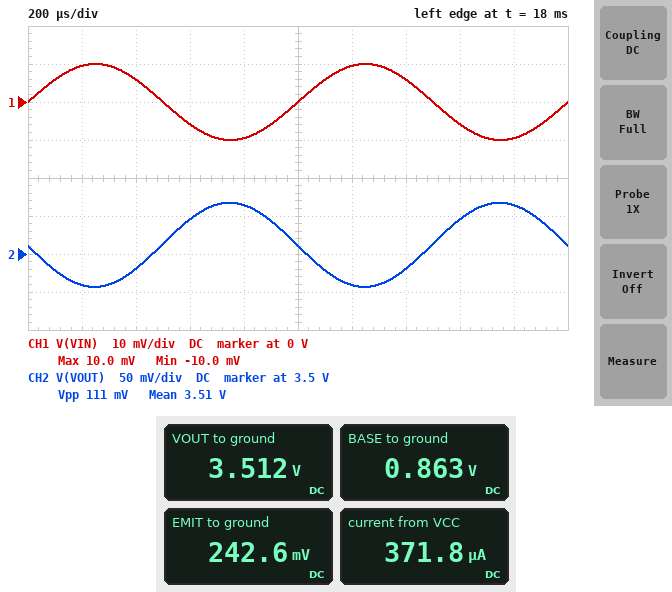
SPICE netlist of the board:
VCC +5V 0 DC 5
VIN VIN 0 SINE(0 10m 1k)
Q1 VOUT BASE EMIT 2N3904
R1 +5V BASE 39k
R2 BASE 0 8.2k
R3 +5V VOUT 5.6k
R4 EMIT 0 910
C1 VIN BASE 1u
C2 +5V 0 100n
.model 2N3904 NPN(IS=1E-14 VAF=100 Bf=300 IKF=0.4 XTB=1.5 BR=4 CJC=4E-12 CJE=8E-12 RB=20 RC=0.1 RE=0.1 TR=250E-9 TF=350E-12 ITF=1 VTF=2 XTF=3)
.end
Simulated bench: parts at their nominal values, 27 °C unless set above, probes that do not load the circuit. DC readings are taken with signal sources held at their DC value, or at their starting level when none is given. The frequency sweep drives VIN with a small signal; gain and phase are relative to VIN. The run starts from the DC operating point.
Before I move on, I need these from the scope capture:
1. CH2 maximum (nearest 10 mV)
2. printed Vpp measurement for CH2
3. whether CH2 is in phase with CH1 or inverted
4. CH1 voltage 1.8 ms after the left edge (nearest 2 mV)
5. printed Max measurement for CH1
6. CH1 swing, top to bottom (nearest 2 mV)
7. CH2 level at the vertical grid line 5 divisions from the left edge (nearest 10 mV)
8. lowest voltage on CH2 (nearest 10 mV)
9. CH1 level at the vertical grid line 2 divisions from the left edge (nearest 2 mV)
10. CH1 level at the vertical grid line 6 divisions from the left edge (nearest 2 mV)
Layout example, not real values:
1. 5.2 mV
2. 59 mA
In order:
1. 3.57 V
2. 111 mV
3. inverted
4. -10 mV
5. 10.0 mV
6. 20 mV
7. 3.51 V
8. 3.46 V
9. 6 mV
10. 10 mV
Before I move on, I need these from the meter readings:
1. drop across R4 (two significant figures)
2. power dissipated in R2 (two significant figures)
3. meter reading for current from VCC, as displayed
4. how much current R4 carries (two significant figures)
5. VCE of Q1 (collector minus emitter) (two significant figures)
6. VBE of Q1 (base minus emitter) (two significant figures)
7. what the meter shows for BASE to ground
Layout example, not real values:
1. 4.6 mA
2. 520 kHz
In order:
1. 240 mV
2. 91 µW
3. 371.8 µA
4. 270 µA
5. 3.3 V
6. 620 mV
7. 0.863 V
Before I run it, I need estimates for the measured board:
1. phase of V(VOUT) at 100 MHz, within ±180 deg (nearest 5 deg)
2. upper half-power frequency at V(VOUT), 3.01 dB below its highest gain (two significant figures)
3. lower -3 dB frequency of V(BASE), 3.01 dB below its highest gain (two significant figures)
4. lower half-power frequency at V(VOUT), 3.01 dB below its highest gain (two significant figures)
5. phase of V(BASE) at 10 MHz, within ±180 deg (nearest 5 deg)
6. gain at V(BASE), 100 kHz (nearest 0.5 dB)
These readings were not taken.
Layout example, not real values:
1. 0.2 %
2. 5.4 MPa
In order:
1. 20 deg
2. 12 MHz
3. 24 Hz
4. 24 Hz
5. 0 deg
6. 0 dB
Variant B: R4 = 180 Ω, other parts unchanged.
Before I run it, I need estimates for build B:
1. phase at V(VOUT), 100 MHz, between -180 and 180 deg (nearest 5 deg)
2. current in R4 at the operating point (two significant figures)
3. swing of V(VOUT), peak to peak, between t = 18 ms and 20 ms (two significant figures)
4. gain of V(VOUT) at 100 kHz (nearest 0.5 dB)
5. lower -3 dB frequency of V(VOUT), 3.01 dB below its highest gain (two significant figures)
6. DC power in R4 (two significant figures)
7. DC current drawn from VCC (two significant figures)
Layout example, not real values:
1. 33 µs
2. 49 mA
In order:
1. 0 deg
2. 860 µA
3. 310 mV
4. 17.0 dB
5. 350 Hz
6. 130 µW
7. 960 µA
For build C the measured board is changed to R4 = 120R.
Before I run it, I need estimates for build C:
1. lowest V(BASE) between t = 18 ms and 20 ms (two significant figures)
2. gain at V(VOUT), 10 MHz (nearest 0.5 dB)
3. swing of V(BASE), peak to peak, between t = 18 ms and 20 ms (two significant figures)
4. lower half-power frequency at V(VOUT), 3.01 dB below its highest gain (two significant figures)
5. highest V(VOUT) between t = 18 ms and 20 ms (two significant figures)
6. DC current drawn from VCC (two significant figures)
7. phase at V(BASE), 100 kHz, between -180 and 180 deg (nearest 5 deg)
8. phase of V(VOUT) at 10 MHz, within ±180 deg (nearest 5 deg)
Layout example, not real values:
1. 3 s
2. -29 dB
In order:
1. 750 mV
2. -1.0 dB
3. 19 mV
4. 520 Hz
5. 460 mV
6. 970 µA
7. 0 deg
8. 10 deg
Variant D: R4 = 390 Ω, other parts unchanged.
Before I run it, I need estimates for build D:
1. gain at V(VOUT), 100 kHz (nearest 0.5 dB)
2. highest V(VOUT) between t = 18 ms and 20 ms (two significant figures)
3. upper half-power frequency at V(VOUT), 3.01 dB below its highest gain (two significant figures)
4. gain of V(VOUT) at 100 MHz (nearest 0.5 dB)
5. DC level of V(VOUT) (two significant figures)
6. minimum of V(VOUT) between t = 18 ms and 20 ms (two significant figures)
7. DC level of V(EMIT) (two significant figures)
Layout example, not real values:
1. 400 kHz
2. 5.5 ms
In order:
1. 22.0 dB
2. 2.0 V
3. 9.1 MHz
4. 4.5 dB
5. 1.9 V
6. 1.8 V
7. 220 mV
